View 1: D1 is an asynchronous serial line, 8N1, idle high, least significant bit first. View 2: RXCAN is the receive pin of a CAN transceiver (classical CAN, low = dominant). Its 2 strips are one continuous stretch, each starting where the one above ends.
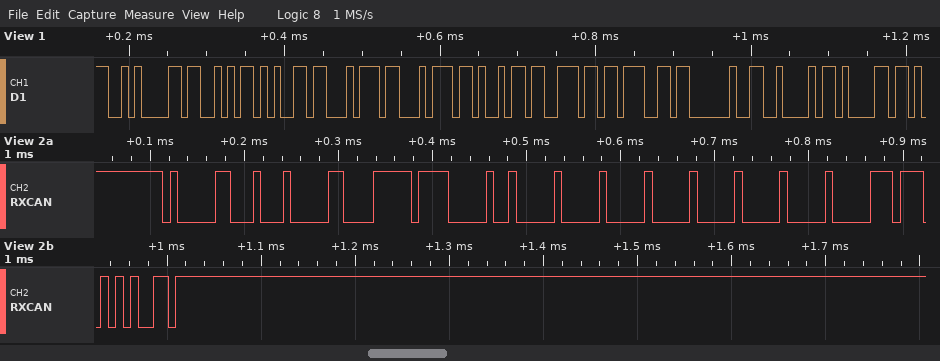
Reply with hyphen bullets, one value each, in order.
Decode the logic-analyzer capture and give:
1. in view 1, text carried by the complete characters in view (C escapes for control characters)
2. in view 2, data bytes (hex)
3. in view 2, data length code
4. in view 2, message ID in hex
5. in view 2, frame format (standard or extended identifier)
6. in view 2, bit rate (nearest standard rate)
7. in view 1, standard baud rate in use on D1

- "\nSetting Ba"
- 21 FF 01 00 00 00 00 00
- 8
- 0x411
- standard
- 125 kbit/s
- 115200 baud
